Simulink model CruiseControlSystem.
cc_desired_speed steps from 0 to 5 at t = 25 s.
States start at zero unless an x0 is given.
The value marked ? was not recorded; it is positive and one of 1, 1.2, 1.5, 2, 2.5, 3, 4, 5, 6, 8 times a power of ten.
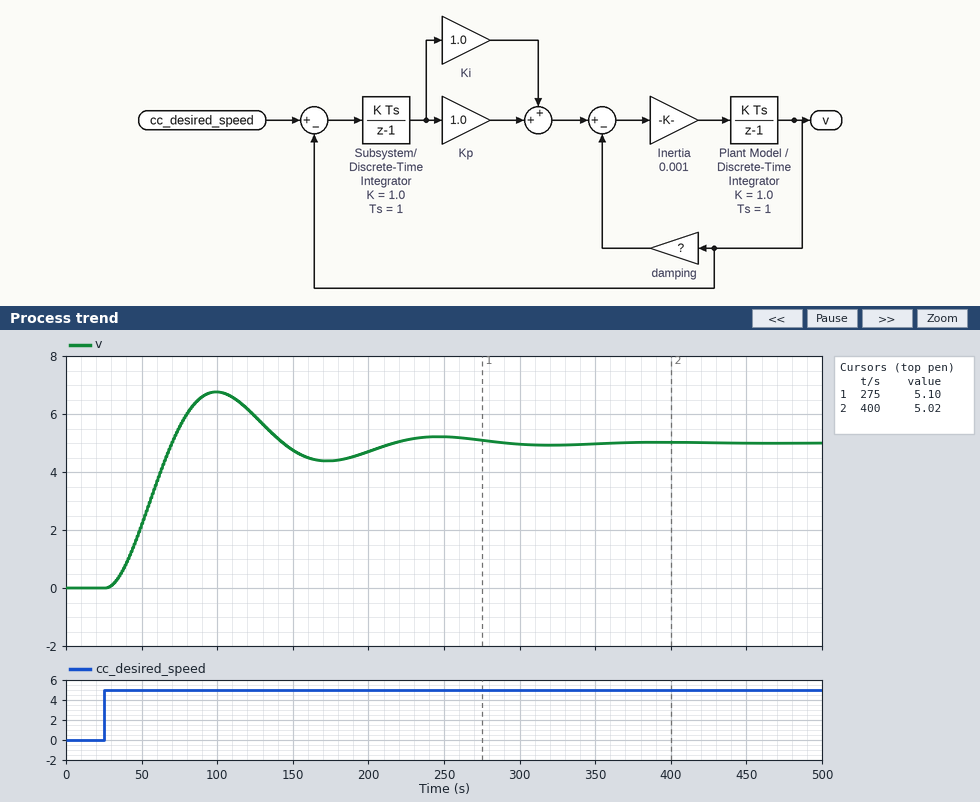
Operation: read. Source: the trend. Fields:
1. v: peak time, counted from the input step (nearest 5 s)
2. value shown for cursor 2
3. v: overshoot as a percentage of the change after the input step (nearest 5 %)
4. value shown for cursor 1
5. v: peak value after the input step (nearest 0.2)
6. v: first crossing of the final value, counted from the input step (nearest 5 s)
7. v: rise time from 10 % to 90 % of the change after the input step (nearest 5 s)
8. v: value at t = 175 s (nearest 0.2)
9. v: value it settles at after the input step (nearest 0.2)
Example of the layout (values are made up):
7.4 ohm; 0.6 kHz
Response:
75 s; 5.02; 35 %; 5.10; 6.8; 45 s; 30 s; 4.4; 5.0
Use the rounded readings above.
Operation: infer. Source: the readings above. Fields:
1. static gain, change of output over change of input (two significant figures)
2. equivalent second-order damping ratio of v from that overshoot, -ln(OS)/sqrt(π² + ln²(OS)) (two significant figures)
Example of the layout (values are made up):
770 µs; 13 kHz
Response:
1.0; 0.32
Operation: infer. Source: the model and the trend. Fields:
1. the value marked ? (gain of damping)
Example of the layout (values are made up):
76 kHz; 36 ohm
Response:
30
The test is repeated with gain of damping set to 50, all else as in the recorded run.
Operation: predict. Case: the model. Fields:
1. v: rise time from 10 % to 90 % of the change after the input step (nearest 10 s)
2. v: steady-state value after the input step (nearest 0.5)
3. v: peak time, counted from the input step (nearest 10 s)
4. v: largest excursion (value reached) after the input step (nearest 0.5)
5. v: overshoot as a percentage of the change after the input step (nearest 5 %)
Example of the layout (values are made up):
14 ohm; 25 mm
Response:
40 s; 5.0; 80 s; 5.5; 15 %
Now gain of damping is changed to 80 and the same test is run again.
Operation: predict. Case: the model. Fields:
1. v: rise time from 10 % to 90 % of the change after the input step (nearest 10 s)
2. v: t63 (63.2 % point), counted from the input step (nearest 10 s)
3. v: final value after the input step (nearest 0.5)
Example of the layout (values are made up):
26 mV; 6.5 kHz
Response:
60 s; 40 s; 5.0
